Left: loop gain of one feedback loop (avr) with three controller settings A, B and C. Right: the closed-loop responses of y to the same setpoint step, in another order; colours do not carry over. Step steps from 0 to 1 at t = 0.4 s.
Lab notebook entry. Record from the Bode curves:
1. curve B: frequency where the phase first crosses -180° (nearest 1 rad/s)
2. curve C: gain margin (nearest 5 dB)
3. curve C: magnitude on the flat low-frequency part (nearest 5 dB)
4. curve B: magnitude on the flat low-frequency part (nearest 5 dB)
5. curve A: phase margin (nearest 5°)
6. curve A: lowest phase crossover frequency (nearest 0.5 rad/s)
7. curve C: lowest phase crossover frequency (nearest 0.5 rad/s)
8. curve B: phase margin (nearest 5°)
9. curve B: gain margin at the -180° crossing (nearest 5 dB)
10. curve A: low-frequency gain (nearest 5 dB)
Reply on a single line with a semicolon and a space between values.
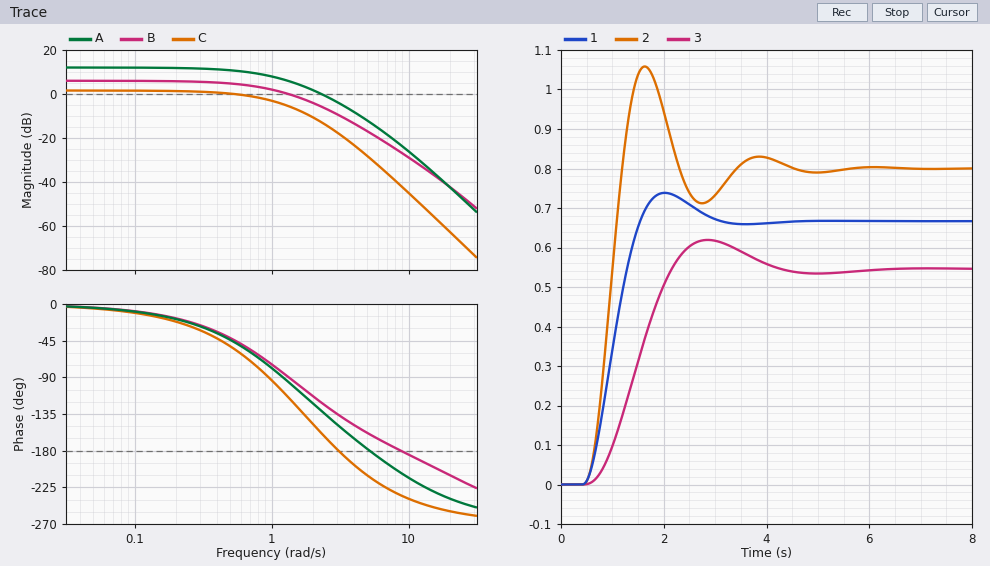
9 rad/s; 20 dB; 0 dB; 5 dB; 50°; 5.0 rad/s; 3.0 rad/s; 90°; 25 dB; 10 dB
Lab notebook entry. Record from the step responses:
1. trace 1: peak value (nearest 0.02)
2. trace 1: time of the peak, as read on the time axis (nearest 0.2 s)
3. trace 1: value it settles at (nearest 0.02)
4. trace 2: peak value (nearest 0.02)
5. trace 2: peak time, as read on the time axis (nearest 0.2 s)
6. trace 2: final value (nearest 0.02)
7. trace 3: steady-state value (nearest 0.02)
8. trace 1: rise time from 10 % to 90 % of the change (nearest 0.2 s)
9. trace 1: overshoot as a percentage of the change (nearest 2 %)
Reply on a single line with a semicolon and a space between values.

0.74; 2.0 s; 0.66; 1.06; 1.6 s; 0.80; 0.54; 0.8 s; 10 %
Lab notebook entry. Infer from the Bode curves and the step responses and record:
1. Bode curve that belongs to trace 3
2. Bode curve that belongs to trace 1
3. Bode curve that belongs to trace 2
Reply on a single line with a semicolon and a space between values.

C; B; A
